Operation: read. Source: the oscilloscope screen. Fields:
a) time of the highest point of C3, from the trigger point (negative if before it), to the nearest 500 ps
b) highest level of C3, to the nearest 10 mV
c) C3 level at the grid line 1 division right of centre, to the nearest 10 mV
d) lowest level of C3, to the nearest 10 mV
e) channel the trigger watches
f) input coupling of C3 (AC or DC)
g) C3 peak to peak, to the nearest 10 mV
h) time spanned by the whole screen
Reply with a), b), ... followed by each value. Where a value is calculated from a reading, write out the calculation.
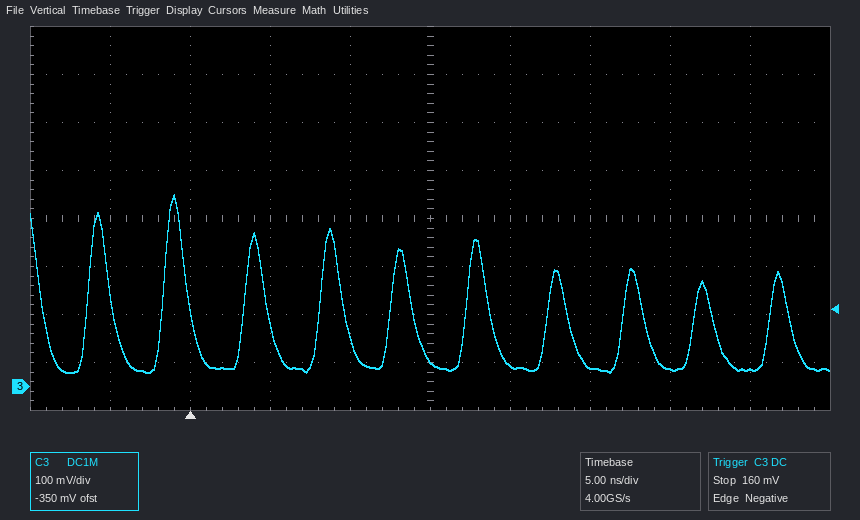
a) -1.0 ns
b) 400 mV
c) 40 mV
d) 30 mV
e) C3
f) DC
g) 400 mV − (30 mV) = 370 mV
h) 50 ns
